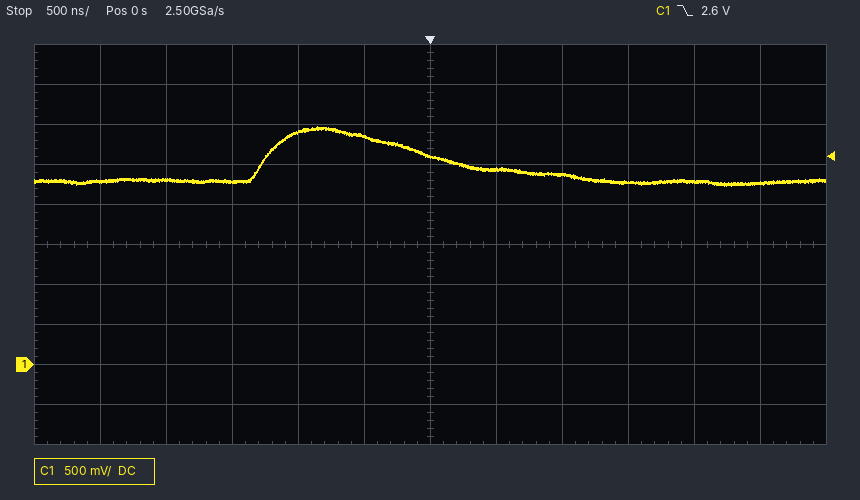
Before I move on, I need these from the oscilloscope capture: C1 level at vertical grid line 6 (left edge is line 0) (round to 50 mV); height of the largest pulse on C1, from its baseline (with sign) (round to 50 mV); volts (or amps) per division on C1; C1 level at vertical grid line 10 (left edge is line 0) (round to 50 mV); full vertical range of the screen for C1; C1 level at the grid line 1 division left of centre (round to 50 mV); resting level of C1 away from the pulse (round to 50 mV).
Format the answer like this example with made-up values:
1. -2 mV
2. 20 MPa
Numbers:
1. 2.60 V
2. +700 mV
3. 500 mV
4. 2.30 V
5. 5 V
6. 2.85 V
7. 2.30 V
